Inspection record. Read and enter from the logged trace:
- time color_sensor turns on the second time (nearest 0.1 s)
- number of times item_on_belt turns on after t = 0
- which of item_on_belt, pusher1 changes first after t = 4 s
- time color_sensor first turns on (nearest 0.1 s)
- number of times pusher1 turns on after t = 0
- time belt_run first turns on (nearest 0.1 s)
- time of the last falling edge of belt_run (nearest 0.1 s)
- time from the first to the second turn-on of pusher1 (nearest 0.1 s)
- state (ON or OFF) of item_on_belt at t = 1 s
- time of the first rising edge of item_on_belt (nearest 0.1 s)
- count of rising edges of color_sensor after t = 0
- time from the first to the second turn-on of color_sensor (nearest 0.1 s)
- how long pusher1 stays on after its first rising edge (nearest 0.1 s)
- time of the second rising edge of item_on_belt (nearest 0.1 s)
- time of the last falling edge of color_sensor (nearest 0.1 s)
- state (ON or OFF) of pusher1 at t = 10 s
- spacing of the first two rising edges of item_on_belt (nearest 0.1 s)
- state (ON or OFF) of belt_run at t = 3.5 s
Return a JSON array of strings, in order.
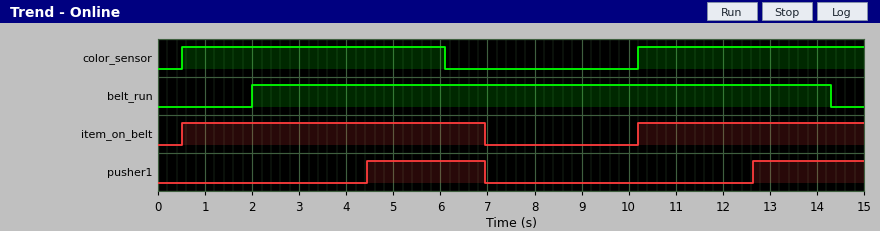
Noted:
["10.2 s", "2", "pusher1", "0.5 s", "2", "2.0 s", "14.3 s", "8.2 s", "ON", "0.5 s", "2", "9.7 s", "2.5 s", "10.2 s", "6.1 s", "OFF", "9.7 s", "ON"]
